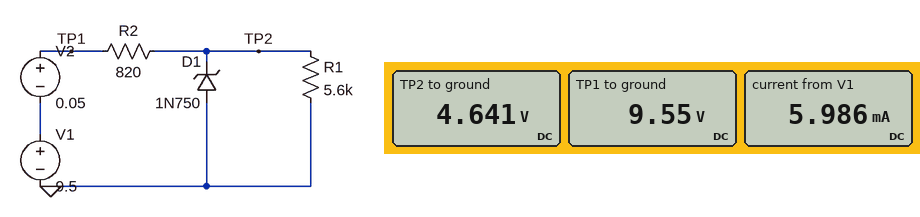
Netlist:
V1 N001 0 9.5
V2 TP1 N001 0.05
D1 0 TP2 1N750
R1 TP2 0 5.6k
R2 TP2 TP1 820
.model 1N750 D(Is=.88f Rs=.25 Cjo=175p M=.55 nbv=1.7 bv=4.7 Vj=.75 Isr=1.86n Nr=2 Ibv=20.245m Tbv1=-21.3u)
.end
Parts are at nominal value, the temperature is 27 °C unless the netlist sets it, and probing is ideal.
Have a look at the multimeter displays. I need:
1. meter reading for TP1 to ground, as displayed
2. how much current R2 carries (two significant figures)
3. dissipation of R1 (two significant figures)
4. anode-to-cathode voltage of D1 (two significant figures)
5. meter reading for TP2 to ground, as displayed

9.55 V
6.0 mA
3.8 mW
-4.6 V
4.641 V
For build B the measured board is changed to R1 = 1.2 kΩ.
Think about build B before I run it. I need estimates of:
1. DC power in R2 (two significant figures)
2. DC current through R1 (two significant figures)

30 mW
3.8 mA
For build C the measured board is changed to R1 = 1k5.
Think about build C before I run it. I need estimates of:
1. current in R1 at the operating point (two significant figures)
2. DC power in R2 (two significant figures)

3.1 mA
30 mW
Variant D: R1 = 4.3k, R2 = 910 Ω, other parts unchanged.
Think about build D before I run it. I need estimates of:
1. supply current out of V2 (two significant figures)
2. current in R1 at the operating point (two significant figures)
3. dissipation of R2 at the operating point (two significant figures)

5.4 mA
1.1 mA
27 mW
